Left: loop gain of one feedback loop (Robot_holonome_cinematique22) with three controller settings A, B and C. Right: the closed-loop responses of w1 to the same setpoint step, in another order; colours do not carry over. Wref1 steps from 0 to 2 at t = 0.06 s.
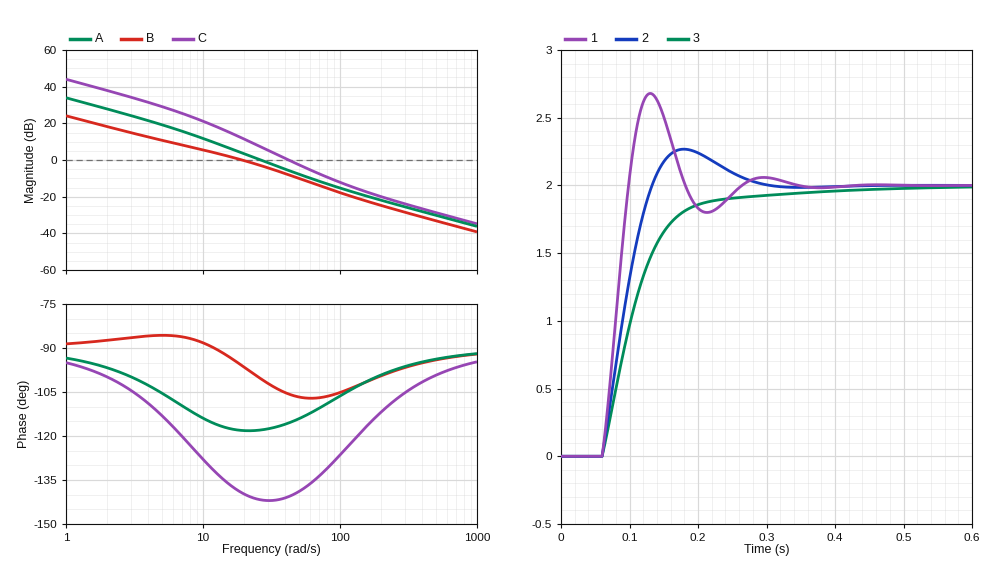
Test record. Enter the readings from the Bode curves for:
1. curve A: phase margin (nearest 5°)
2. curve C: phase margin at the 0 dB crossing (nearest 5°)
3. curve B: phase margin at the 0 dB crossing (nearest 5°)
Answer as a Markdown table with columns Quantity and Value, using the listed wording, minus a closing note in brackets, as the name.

| Quantity | Value |
|---|---|
| curve A: phase margin | 60° |
| curve C: phase margin at the 0 dB crossing | 40° |
| curve B: phase margin at the 0 dB crossing | 85° |
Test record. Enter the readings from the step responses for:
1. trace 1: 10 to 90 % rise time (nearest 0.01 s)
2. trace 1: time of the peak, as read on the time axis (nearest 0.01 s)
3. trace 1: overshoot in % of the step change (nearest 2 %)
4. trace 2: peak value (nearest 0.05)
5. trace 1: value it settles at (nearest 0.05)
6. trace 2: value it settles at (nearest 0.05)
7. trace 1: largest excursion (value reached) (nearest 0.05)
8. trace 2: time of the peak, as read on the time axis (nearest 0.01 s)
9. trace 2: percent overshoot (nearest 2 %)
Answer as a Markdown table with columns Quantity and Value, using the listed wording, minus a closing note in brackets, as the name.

| Quantity | Value |
|---|---|
| trace 1: 10 to 90 % rise time | 0.03 s |
| trace 1: time of the peak, as read on the time axis | 0.13 s |
| trace 1: overshoot in % of the step change | 34 % |
| trace 2: peak value | 2.25 |
| trace 1: value it settles at | 2.00 |
| trace 2: value it settles at | 2.00 |
| trace 1: largest excursion (value reached) | 2.70 |
| trace 2: time of the peak, as read on the time axis | 0.18 s |
| trace 2: percent overshoot | 14 % |
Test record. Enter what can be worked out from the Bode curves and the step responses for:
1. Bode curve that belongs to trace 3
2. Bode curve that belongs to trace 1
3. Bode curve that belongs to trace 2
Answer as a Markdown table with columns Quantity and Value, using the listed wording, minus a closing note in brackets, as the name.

| Quantity | Value |
|---|---|
| Bode curve that belongs to trace 3 | B |
| Bode curve that belongs to trace 1 | C |
| Bode curve that belongs to trace 2 | A |
